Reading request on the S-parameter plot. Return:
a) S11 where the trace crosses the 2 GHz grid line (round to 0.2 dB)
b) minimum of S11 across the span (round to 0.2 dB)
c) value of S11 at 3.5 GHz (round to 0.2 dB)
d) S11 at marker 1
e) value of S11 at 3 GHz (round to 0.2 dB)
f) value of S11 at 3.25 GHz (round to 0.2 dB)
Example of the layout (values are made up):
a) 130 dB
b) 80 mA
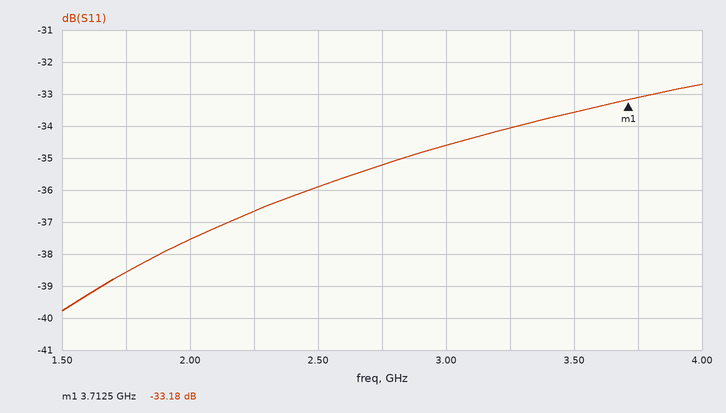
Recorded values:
a) -37.6 dB
b) -39.8 dB
c) -33.6 dB
d) -33.18 dB
e) -34.6 dB
f) -34.0 dB
